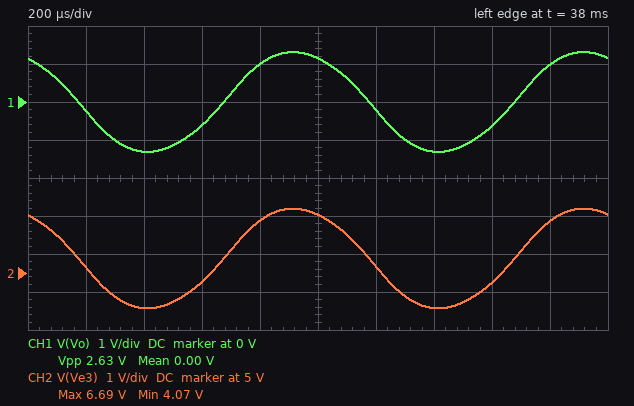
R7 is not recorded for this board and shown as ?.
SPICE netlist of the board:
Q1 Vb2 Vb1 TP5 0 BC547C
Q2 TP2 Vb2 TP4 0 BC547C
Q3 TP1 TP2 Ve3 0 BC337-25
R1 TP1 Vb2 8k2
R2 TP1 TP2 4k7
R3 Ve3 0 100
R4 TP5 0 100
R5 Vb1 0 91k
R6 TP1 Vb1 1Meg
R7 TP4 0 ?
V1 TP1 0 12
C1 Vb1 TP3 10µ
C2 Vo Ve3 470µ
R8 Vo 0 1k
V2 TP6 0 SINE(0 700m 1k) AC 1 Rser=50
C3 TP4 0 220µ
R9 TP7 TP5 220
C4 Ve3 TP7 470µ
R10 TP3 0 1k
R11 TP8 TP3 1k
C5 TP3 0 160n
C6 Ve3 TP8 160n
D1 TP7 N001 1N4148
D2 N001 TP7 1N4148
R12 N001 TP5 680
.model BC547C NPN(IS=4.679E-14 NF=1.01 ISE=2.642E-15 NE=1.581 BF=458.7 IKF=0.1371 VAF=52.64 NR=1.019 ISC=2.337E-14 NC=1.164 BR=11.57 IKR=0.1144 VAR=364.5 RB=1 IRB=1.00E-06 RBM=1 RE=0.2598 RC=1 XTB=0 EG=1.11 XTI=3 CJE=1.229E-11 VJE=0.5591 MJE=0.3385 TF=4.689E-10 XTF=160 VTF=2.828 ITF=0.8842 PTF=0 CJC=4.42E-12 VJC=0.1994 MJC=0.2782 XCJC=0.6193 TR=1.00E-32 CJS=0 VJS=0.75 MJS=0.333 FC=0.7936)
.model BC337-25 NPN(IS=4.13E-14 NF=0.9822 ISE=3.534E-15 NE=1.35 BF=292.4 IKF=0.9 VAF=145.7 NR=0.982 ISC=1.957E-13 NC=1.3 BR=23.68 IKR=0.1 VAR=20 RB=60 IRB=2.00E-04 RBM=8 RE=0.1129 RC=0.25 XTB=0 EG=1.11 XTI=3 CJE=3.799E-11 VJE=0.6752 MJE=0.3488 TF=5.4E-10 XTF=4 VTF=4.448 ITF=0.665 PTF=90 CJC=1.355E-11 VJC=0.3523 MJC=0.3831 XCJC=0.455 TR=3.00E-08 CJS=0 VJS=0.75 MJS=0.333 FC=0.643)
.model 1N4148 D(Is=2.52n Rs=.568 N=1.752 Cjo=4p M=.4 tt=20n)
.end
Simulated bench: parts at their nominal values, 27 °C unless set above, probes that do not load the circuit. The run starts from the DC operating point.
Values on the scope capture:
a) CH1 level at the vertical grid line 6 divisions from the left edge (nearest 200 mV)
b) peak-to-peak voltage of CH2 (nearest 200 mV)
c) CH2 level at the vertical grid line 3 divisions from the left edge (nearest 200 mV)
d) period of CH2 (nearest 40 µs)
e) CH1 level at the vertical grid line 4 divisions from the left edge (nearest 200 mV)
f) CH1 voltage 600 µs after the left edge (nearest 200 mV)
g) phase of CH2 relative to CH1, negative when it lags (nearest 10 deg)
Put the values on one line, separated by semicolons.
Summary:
-200 mV; 2.6 V; 4.8 V; 1.00 ms; 1.0 V; -600 mV; 0 deg
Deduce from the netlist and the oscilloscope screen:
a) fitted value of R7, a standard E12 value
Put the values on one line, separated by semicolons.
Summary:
560 Ω
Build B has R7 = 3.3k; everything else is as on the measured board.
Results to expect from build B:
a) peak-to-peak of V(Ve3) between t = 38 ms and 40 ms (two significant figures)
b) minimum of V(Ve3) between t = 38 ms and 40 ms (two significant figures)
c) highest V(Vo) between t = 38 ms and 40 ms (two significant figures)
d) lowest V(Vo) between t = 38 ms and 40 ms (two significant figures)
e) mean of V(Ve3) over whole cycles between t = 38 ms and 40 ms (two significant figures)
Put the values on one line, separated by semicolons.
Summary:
1.6 V; 7.9 V; 710 mV; -890 mV; 8.7 V
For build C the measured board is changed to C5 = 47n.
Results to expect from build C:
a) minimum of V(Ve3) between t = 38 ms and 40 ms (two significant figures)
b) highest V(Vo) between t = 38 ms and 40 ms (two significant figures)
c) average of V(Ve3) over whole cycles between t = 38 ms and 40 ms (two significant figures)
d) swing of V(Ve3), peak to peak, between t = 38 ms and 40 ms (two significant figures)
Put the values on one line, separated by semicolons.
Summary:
1.7 V; 3.0 V; 4.3 V; 6.7 V
